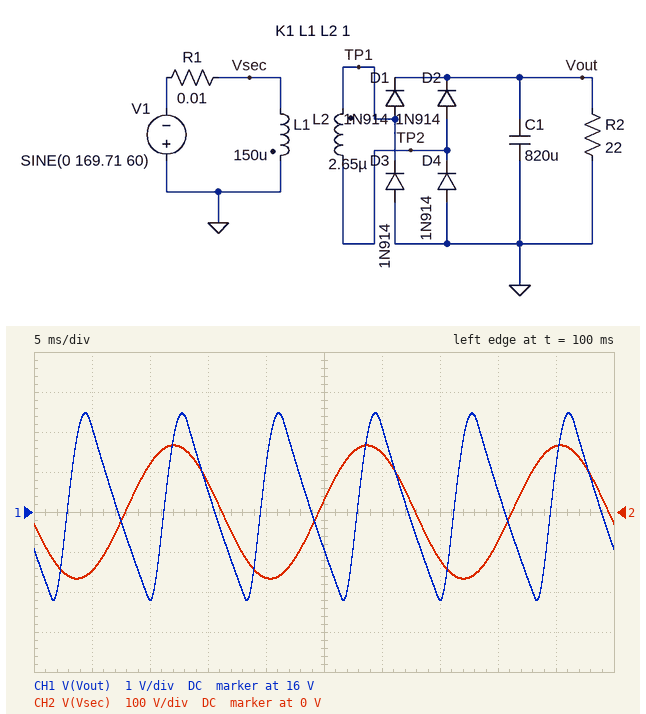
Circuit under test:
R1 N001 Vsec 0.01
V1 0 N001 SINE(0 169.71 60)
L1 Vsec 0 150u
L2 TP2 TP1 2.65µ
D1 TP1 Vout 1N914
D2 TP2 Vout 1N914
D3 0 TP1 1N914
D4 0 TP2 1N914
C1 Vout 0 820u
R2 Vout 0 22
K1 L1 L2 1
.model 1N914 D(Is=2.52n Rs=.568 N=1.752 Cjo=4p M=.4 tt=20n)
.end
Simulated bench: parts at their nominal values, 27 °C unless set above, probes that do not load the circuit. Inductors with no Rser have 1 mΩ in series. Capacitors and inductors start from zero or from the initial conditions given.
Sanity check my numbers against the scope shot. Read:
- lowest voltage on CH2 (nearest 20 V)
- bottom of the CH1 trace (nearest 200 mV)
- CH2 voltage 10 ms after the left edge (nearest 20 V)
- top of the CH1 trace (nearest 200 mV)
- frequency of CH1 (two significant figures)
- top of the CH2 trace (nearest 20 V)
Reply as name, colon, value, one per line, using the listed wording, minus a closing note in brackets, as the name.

lowest voltage on CH2: -160 V
bottom of the CH1 trace: 13.8 V
CH2 voltage 10 ms after the left edge: 120 V
top of the CH1 trace: 18.4 V
frequency of CH1: 120 Hz
top of the CH2 trace: 160 V
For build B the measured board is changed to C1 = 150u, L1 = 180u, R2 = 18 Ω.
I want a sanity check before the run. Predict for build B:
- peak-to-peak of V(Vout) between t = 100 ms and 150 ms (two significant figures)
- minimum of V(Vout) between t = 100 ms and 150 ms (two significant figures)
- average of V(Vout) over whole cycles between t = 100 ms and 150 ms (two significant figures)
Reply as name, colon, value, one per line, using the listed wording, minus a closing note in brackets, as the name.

peak-to-peak of V(Vout) between t = 100 ms and 150 ms: 13 V
minimum of V(Vout) between t = 100 ms and 150 ms: 4.4 V
average of V(Vout) over whole cycles between t = 100 ms and 150 ms: 12 V
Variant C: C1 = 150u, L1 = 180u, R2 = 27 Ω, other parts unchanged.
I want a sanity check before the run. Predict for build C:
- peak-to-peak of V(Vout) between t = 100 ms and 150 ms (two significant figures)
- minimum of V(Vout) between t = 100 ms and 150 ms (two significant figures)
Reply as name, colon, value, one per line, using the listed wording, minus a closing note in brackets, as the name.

peak-to-peak of V(Vout) between t = 100 ms and 150 ms: 12 V
minimum of V(Vout) between t = 100 ms and 150 ms: 6.2 V
